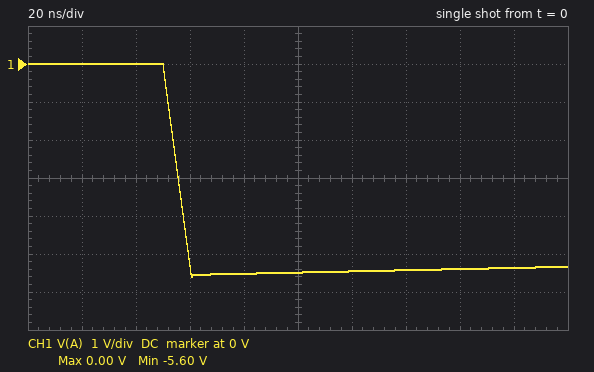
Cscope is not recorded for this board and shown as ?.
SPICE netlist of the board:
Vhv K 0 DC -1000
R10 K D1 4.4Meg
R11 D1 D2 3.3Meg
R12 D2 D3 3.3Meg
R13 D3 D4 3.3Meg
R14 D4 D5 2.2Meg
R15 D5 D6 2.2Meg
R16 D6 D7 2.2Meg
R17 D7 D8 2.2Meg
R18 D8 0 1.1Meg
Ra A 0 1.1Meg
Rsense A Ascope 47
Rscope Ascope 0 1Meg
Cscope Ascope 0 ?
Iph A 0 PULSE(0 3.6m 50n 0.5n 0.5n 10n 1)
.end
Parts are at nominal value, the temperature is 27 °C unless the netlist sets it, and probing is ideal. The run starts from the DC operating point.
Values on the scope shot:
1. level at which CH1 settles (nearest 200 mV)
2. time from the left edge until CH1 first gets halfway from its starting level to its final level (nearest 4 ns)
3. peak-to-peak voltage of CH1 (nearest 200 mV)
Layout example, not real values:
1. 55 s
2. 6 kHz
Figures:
1. -5.4 V
2. 56 ns
3. 5.6 V
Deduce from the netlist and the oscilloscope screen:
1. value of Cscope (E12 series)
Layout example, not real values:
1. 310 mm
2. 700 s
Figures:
1. 6.8 pF
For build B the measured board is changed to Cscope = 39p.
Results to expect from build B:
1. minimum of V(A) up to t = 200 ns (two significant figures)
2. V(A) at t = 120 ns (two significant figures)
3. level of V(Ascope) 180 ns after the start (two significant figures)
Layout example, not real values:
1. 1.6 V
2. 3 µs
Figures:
1. -1.1 V
2. -970 mV
3. -960 mV
